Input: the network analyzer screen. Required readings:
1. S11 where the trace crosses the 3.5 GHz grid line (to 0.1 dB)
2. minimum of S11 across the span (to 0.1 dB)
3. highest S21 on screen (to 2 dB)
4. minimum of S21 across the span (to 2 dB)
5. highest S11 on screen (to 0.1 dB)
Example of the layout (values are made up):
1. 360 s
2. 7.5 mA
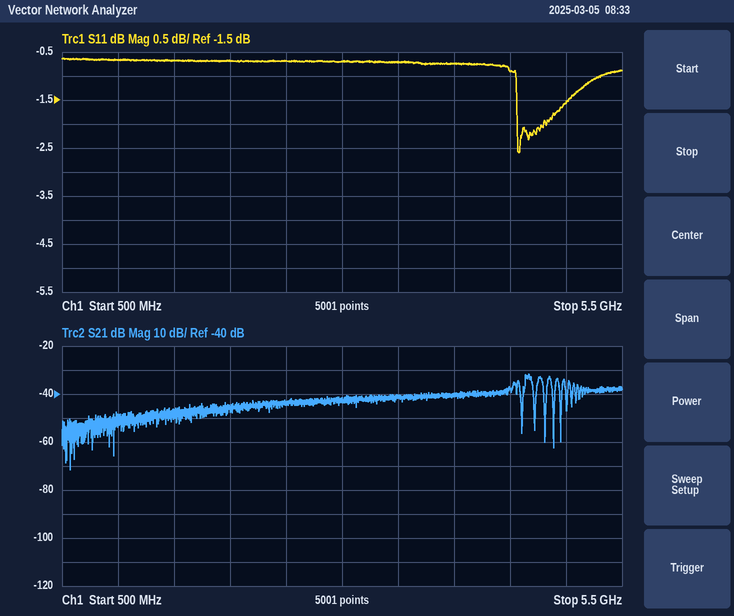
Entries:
1. -0.7 dB
2. -2.6 dB
3. -32 dB
4. -72 dB
5. -0.6 dB
